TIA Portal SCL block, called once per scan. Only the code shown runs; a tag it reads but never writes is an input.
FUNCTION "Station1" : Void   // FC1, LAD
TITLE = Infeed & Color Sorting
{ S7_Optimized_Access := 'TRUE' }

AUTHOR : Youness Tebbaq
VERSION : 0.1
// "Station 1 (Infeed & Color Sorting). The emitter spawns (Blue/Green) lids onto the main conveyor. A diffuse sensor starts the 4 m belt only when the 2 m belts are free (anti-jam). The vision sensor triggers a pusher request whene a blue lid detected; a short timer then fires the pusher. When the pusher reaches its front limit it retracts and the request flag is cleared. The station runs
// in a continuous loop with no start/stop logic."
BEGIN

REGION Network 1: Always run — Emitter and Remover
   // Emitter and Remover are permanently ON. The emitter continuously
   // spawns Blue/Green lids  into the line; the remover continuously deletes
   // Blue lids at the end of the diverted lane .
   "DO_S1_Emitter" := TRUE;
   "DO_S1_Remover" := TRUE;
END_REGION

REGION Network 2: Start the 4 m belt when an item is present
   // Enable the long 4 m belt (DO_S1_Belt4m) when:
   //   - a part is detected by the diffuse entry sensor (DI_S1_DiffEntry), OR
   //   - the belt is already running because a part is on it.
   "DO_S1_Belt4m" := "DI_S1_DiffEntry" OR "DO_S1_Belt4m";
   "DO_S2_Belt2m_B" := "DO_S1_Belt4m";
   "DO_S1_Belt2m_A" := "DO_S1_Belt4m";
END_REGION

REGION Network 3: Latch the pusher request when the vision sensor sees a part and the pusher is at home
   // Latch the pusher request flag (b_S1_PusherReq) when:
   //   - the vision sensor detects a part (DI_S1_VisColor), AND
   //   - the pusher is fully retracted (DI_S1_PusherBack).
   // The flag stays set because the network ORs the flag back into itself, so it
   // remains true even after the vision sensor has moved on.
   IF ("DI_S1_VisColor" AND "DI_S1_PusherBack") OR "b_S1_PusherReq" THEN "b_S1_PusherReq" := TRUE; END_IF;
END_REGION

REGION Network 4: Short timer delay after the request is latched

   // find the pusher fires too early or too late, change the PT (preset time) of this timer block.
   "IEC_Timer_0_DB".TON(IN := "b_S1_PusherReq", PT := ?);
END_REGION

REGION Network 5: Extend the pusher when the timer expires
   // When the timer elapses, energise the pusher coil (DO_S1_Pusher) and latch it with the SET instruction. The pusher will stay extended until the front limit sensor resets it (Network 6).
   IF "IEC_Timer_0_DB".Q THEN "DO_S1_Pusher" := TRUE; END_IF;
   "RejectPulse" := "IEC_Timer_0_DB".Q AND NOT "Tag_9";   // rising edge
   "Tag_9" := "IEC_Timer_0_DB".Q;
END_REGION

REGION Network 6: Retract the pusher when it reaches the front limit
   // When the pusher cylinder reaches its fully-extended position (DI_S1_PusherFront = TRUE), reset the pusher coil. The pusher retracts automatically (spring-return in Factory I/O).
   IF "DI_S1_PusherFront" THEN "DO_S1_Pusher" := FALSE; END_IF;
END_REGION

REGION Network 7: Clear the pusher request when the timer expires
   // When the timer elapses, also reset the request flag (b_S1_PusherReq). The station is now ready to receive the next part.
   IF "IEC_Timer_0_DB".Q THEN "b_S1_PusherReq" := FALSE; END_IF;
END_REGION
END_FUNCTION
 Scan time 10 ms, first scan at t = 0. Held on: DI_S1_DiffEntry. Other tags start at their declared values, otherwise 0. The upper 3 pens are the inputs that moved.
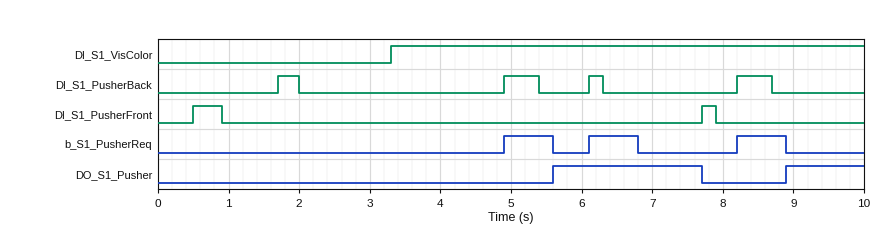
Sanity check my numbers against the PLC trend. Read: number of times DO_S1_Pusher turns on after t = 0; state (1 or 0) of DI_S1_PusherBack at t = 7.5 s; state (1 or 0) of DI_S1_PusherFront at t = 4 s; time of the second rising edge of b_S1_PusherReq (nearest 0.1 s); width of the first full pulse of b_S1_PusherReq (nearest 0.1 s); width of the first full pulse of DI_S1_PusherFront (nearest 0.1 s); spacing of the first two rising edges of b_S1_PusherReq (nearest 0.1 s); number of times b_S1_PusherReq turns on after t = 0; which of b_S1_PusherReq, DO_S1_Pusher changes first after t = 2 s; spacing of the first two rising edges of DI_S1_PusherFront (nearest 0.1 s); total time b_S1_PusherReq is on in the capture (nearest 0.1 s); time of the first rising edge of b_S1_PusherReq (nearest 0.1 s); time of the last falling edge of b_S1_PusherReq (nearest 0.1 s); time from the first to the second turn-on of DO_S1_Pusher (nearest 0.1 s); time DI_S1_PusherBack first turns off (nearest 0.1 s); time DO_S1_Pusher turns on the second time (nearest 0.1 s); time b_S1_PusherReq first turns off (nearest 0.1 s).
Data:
2
0
0
6.1 s
0.7 s
0.4 s
1.2 s
3
b_S1_PusherReq
7.2 s
2.1 s
4.9 s
8.9 s
3.3 s
2.0 s
8.9 s
5.6 s
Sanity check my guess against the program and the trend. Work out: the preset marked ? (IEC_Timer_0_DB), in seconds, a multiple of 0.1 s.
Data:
0.7 s
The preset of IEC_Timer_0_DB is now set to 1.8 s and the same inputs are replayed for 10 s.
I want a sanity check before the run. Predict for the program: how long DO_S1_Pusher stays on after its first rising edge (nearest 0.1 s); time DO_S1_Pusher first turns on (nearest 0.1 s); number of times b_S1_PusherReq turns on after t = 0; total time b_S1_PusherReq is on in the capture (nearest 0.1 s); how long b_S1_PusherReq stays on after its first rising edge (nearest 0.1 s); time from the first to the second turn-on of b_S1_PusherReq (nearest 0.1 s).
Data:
1.0 s
6.7 s
2
3.6 s
1.8 s
3.3 s
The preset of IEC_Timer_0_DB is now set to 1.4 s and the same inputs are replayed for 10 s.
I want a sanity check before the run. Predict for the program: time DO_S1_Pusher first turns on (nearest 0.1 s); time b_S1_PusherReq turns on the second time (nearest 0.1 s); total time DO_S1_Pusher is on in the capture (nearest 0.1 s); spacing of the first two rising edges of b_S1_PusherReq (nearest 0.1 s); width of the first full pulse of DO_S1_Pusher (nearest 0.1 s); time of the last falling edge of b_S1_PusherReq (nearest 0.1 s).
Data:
6.3 s
8.2 s
1.8 s
3.3 s
1.4 s
9.6 s
